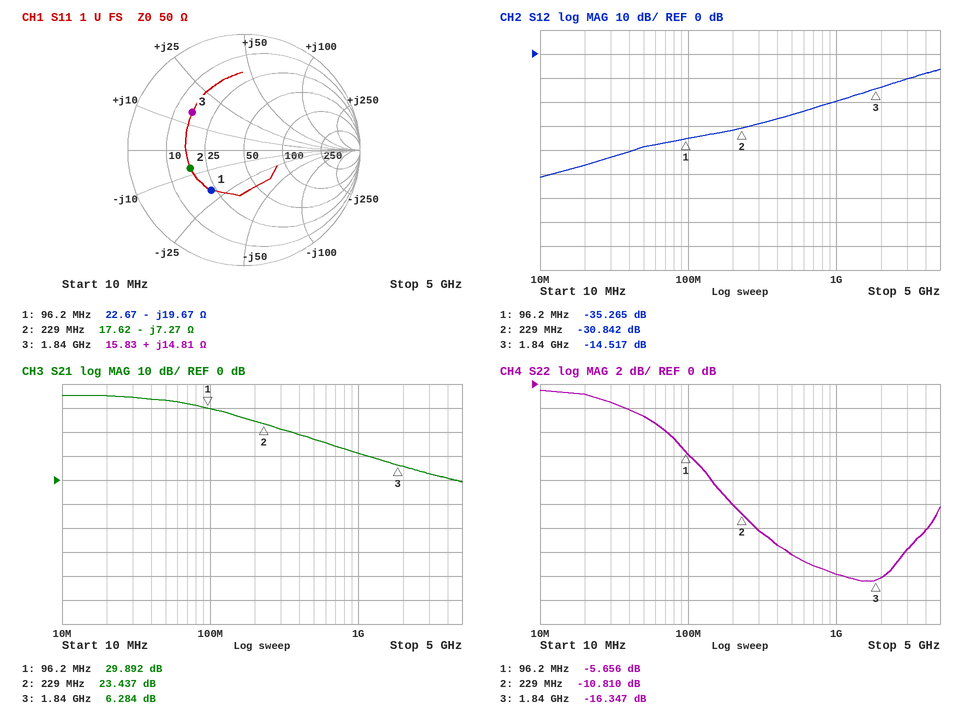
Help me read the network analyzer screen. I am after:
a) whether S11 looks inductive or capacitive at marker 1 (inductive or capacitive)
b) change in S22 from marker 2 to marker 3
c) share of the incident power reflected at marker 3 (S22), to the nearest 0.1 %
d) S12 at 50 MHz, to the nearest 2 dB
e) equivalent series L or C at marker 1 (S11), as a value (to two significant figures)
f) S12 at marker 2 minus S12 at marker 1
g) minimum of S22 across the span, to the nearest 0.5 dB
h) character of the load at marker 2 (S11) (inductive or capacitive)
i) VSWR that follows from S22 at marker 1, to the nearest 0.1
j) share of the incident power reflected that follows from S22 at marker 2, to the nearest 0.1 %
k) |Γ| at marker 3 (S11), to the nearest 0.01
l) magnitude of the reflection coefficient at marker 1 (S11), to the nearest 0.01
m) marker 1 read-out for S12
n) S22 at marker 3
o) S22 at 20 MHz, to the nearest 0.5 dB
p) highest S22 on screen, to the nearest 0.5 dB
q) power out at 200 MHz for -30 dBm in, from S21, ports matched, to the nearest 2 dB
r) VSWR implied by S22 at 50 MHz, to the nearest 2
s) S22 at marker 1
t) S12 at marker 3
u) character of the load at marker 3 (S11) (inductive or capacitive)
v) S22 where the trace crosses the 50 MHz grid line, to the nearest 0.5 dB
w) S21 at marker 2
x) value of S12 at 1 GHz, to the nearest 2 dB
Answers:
capacitive
-5.537 dB
2.3 %
-38 dB
84 pF
4.423 dB
-16.5 dB
capacitive
3.2
8.3 %
0.55
0.45
-35.265 dB
-16.347 dB
-1.0 dB
-0.5 dB
-6 dBm
6
-5.656 dB
-14.517 dB
inductive
-2.5 dB
23.437 dB
-20 dB
